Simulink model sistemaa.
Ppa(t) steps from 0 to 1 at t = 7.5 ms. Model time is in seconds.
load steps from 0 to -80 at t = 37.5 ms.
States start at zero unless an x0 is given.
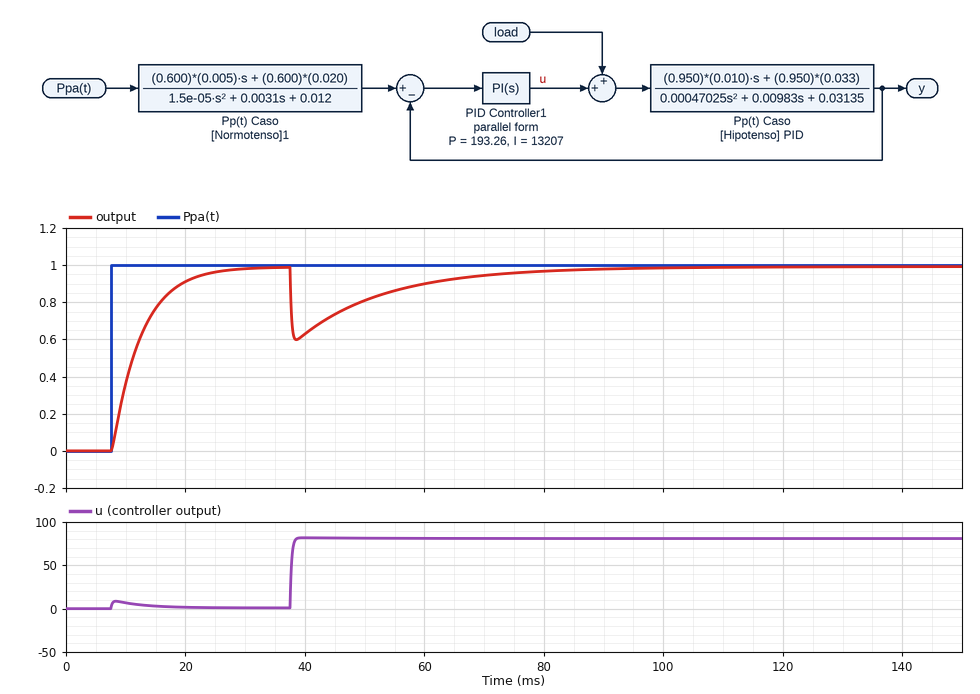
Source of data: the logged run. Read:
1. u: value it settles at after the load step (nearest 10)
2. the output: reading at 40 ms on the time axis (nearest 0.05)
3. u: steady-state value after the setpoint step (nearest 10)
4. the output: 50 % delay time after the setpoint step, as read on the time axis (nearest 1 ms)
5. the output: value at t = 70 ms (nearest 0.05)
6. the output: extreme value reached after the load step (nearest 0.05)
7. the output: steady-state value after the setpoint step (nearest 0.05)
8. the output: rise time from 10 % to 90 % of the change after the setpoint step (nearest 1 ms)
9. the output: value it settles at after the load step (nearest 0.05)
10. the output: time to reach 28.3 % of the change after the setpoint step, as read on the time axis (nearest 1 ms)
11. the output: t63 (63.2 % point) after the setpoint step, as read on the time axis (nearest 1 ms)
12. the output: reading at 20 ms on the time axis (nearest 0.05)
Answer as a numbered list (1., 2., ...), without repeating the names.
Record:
1. 80
2. 0.65
3. 0
4. 11 ms
5. 0.95
6. 0.60
7. 1.00
8. 11 ms
9. 1.00
10. 9 ms
11. 13 ms
12. 0.90
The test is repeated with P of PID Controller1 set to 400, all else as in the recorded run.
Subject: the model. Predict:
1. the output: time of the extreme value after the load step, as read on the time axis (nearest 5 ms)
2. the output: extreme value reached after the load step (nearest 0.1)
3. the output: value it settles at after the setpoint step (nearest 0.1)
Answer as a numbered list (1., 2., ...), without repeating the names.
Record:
1. 40 ms
2. 0.8
3. 1.0
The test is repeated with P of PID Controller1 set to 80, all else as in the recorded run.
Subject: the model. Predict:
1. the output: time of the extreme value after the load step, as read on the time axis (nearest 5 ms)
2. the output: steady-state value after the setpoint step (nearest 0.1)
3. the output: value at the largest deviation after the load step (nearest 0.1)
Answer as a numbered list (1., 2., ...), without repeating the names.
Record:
1. 40 ms
2. 1.0
3. 0.2
